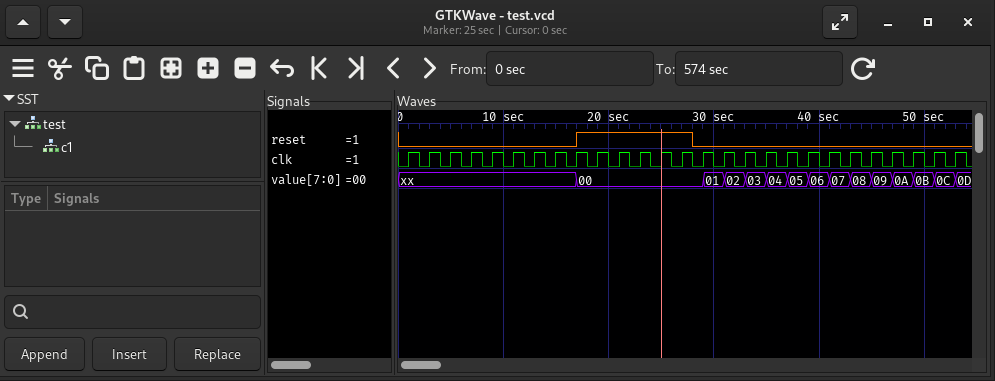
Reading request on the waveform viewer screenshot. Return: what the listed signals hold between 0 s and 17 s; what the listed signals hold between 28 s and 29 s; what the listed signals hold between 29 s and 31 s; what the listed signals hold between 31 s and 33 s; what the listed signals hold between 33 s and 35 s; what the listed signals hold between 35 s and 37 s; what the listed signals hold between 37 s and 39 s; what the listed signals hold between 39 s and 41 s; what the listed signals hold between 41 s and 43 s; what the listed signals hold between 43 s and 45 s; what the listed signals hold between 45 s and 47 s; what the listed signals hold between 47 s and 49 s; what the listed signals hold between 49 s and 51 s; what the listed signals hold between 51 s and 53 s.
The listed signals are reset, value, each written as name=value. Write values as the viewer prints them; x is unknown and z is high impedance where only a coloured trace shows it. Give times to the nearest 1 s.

reset=0, value=xx
reset=0, value=00
reset=0, value=01
reset=0, value=02
reset=0, value=03
reset=0, value=04
reset=0, value=05
reset=0, value=06
reset=0, value=07
reset=0, value=08
reset=0, value=09
reset=0, value=0A
reset=0, value=0B
reset=0, value=0C
